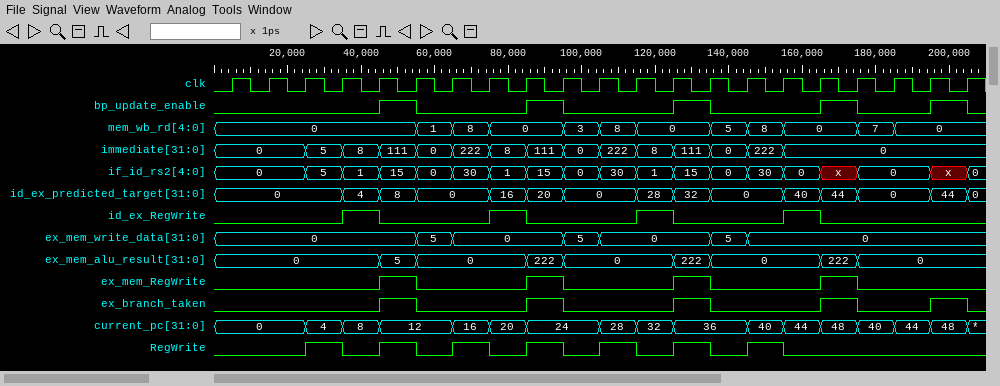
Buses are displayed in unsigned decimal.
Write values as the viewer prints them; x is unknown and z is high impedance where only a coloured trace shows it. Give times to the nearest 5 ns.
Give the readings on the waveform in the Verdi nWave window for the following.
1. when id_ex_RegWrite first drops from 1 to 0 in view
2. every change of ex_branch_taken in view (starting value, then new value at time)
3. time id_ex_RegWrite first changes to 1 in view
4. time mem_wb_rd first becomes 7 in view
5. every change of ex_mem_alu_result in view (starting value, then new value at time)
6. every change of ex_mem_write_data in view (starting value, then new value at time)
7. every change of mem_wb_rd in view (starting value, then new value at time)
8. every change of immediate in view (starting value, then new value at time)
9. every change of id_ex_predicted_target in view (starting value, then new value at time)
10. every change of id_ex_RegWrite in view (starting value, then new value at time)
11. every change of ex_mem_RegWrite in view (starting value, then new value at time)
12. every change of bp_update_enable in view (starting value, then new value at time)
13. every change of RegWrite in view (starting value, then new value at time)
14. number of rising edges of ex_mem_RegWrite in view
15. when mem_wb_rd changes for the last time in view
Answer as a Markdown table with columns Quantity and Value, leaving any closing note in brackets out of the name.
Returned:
| Quantity | Value |
|---|---|
| when id_ex_RegWrite first drops from 1 to 0 in view | 45 ns |
| every change of ex_branch_taken in view | 0, 1 at 45 ns, 0 at 55 ns, 1 at 85 ns, 0 at 95 ns, 1 at 125 ns, 0 at 135 ns, 1 at 165 ns, 0 at 175 ns, 1 at 195 ns, 0 at 205 ns |
| time id_ex_RegWrite first changes to 1 in view | 35 ns |
| time mem_wb_rd first becomes 7 in view | 175 ns |
| every change of ex_mem_alu_result in view | 0, 5 at 45 ns, 0 at 55 ns, 222 at 85 ns, 0 at 95 ns, 222 at 125 ns, 0 at 135 ns, 222 at 165 ns, 0 at 175 ns |
| every change of ex_mem_write_data in view | 0, 5 at 55 ns, 0 at 65 ns, 5 at 95 ns, 0 at 105 ns, 5 at 135 ns, 0 at 145 ns |
| every change of mem_wb_rd in view | 0, 1 at 55 ns, 8 at 65 ns, 0 at 75 ns, 3 at 95 ns, 8 at 105 ns, 0 at 115 ns, 5 at 135 ns, 8 at 145 ns, 0 at 155 ns, 7 at 175 ns, 0 at 185 ns |
| every change of immediate in view | 0, 5 at 25 ns, 8 at 35 ns, 111 at 45 ns, 0 at 55 ns, 222 at 65 ns, 8 at 75 ns, 111 at 85 ns, 0 at 95 ns, 222 at 105 ns, 8 at 115 ns, 111 at 125 ns, 0 at 135 ns, 222 at 145 ns, 0 at 155 ns |
| every change of id_ex_predicted_target in view | 0, 4 at 35 ns, 8 at 45 ns, 0 at 55 ns, 16 at 75 ns, 20 at 85 ns, 0 at 95 ns, 28 at 115 ns, 32 at 125 ns, 0 at 135 ns, 40 at 155 ns, 44 at 165 ns, 0 at 175 ns, 44 at 195 ns, 0 at 205 ns |
| every change of id_ex_RegWrite in view | 0, 1 at 35 ns, 0 at 45 ns, 1 at 75 ns, 0 at 85 ns, 1 at 115 ns, 0 at 125 ns, 1 at 155 ns, 0 at 165 ns |
| every change of ex_mem_RegWrite in view | 0, 1 at 45 ns, 0 at 55 ns, 1 at 85 ns, 0 at 95 ns, 1 at 125 ns, 0 at 135 ns, 1 at 165 ns, 0 at 175 ns |
| every change of bp_update_enable in view | 0, 1 at 45 ns, 0 at 55 ns, 1 at 85 ns, 0 at 95 ns, 1 at 125 ns, 0 at 135 ns, 1 at 165 ns, 0 at 175 ns, 1 at 195 ns, 0 at 205 ns |
| every change of RegWrite in view | 0, 1 at 25 ns, 0 at 35 ns, 1 at 45 ns, 0 at 55 ns, 1 at 65 ns, 0 at 75 ns, 1 at 85 ns, 0 at 95 ns, 1 at 105 ns, 0 at 115 ns, 1 at 125 ns, 0 at 135 ns, 1 at 145 ns, 0 at 155 ns |
| number of rising edges of ex_mem_RegWrite in view | 4 |
| when mem_wb_rd changes for the last time in view | 185 ns |
